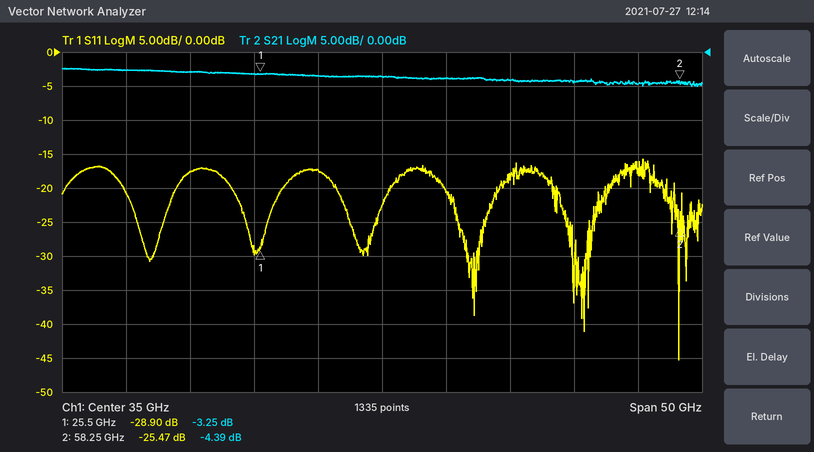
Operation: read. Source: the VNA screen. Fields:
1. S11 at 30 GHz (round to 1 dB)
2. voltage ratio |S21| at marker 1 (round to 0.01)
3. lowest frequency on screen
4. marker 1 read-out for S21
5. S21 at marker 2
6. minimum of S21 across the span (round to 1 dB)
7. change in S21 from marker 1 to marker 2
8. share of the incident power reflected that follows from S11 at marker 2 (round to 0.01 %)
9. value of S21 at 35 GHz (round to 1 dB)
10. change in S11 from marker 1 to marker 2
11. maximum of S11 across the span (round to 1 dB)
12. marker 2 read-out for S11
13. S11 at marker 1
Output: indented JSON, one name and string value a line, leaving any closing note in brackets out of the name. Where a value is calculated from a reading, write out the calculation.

{
  "S11 at 30 GHz": "-17 dB",
  "voltage ratio |S21| at marker 1": "10^(-3.25/20) ≈ 0.69",
  "lowest frequency on screen": "10 GHz",
  "marker 1 read-out for S21": "-3.25 dB",
  "S21 at marker 2": "-4.39 dB",
  "minimum of S21 across the span": "-5 dB",
  "change in S21 from marker 1 to marker 2": "-4.39 − (-3.25) = -1.14 dB",
  "share of the incident power reflected that follows from S11 at marker 2": "10^(-25.47/10) ≈ 0.28 %",
  "value of S21 at 35 GHz": "-4 dB",
  "change in S11 from marker 1 to marker 2": "-25.47 − (-28.9) = 3.43 dB",
  "maximum of S11 across the span": "-16 dB",
  "marker 2 read-out for S11": "-25.47 dB",
  "S11 at marker 1": "-28.90 dB"
}
